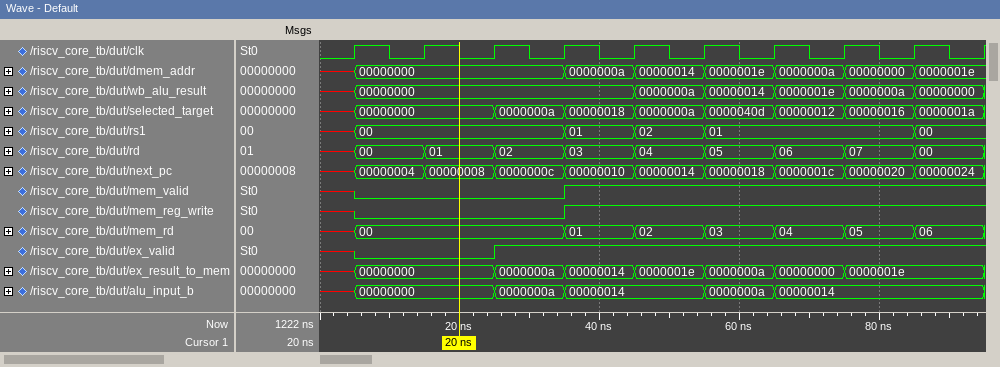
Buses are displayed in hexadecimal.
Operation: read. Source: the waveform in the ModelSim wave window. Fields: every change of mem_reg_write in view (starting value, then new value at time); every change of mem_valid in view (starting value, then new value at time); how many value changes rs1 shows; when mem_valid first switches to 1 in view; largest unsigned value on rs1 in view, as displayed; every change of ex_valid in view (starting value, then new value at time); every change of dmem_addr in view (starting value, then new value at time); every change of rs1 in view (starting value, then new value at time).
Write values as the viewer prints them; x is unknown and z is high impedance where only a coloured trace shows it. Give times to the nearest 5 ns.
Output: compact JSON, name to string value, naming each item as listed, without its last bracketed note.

{"every change of mem_reg_write in view": "x, 0 at 5 ns, 1 at 35 ns", "every change of mem_valid in view": "x, 0 at 5 ns, 1 at 35 ns", "how many value changes rs1 shows": "5", "when mem_valid first switches to 1 in view": "35 ns", "largest unsigned value on rs1 in view, as displayed": "02", "every change of ex_valid in view": "x, 0 at 5 ns, 1 at 25 ns", "every change of dmem_addr in view": "x, 00000000 at 5 ns, 0000000a at 35 ns, 00000014 at 45 ns, 0000001e at 55 ns, 0000000a at 65 ns, 00000000 at 75 ns, 0000001e at 85 ns", "every change of rs1 in view": "x, 00 at 5 ns, 01 at 35 ns, 02 at 45 ns, 01 at 55 ns, 00 at 85 ns"}
